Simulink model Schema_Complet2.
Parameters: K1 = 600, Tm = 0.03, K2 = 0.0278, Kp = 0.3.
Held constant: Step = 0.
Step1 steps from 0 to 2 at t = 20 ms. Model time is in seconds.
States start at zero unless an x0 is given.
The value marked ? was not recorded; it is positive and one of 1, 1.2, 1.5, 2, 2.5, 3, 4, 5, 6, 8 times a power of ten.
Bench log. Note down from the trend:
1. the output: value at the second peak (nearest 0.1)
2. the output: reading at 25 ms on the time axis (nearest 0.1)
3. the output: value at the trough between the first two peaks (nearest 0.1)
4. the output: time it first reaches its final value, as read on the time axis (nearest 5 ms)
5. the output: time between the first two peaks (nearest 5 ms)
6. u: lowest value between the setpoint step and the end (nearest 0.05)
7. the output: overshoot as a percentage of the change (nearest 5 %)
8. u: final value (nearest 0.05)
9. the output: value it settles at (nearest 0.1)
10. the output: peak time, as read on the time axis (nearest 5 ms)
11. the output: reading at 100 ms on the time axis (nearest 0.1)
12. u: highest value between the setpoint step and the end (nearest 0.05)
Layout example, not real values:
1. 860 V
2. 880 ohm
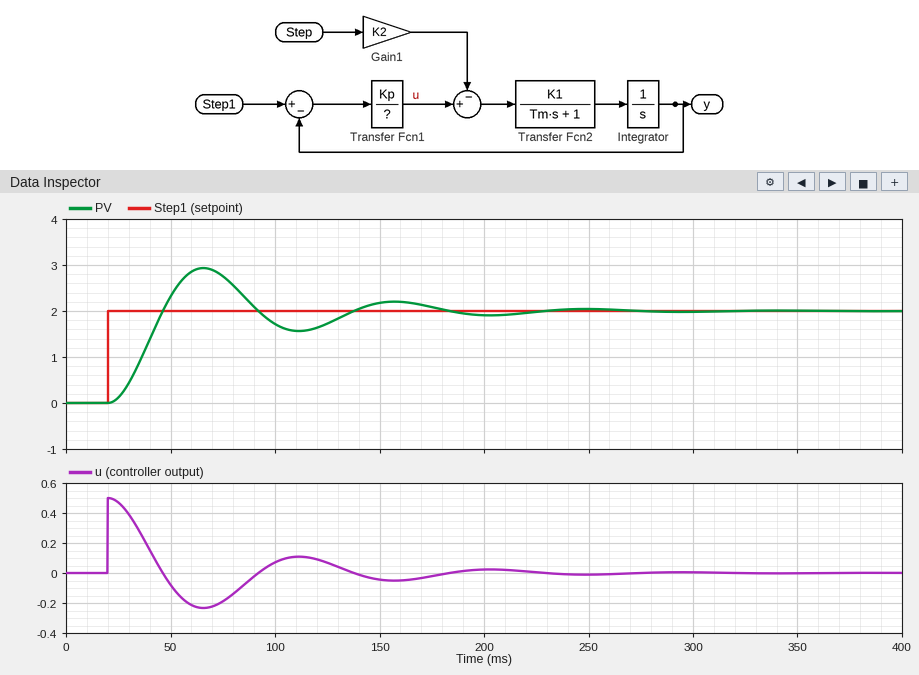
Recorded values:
1. 2.2
2. 0.1
3. 1.6
4. 45 ms
5. 90 ms
6. -0.25
7. 45 %
8. 0.00
9. 2.0
10. 65 ms
11. 1.7
12. 0.50
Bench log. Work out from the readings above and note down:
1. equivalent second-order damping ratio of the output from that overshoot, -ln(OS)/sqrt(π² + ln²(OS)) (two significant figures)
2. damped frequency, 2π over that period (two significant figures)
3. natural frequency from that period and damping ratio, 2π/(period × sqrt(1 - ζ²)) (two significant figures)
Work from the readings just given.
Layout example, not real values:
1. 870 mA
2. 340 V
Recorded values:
1. 0.25
2. 0.070 rad/ms
3. 0.072 rad/ms
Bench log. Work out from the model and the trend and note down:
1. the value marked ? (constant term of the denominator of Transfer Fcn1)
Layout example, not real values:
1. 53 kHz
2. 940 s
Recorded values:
1. 1.2
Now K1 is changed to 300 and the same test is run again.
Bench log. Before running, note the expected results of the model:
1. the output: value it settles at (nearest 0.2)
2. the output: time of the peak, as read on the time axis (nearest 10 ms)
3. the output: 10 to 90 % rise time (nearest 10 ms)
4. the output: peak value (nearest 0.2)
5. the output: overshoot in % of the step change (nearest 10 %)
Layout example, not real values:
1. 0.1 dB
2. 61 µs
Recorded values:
1. 2.0
2. 90 ms
3. 30 ms
4. 2.6
5. 30 %
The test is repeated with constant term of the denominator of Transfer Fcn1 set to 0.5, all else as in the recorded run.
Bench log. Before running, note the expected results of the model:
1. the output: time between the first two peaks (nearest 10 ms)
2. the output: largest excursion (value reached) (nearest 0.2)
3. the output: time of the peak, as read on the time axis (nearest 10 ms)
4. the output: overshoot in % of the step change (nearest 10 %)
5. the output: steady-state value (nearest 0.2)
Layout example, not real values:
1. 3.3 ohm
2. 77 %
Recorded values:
1. 60 ms
2. 3.2
3. 50 ms
4. 60 %
5. 2.0
